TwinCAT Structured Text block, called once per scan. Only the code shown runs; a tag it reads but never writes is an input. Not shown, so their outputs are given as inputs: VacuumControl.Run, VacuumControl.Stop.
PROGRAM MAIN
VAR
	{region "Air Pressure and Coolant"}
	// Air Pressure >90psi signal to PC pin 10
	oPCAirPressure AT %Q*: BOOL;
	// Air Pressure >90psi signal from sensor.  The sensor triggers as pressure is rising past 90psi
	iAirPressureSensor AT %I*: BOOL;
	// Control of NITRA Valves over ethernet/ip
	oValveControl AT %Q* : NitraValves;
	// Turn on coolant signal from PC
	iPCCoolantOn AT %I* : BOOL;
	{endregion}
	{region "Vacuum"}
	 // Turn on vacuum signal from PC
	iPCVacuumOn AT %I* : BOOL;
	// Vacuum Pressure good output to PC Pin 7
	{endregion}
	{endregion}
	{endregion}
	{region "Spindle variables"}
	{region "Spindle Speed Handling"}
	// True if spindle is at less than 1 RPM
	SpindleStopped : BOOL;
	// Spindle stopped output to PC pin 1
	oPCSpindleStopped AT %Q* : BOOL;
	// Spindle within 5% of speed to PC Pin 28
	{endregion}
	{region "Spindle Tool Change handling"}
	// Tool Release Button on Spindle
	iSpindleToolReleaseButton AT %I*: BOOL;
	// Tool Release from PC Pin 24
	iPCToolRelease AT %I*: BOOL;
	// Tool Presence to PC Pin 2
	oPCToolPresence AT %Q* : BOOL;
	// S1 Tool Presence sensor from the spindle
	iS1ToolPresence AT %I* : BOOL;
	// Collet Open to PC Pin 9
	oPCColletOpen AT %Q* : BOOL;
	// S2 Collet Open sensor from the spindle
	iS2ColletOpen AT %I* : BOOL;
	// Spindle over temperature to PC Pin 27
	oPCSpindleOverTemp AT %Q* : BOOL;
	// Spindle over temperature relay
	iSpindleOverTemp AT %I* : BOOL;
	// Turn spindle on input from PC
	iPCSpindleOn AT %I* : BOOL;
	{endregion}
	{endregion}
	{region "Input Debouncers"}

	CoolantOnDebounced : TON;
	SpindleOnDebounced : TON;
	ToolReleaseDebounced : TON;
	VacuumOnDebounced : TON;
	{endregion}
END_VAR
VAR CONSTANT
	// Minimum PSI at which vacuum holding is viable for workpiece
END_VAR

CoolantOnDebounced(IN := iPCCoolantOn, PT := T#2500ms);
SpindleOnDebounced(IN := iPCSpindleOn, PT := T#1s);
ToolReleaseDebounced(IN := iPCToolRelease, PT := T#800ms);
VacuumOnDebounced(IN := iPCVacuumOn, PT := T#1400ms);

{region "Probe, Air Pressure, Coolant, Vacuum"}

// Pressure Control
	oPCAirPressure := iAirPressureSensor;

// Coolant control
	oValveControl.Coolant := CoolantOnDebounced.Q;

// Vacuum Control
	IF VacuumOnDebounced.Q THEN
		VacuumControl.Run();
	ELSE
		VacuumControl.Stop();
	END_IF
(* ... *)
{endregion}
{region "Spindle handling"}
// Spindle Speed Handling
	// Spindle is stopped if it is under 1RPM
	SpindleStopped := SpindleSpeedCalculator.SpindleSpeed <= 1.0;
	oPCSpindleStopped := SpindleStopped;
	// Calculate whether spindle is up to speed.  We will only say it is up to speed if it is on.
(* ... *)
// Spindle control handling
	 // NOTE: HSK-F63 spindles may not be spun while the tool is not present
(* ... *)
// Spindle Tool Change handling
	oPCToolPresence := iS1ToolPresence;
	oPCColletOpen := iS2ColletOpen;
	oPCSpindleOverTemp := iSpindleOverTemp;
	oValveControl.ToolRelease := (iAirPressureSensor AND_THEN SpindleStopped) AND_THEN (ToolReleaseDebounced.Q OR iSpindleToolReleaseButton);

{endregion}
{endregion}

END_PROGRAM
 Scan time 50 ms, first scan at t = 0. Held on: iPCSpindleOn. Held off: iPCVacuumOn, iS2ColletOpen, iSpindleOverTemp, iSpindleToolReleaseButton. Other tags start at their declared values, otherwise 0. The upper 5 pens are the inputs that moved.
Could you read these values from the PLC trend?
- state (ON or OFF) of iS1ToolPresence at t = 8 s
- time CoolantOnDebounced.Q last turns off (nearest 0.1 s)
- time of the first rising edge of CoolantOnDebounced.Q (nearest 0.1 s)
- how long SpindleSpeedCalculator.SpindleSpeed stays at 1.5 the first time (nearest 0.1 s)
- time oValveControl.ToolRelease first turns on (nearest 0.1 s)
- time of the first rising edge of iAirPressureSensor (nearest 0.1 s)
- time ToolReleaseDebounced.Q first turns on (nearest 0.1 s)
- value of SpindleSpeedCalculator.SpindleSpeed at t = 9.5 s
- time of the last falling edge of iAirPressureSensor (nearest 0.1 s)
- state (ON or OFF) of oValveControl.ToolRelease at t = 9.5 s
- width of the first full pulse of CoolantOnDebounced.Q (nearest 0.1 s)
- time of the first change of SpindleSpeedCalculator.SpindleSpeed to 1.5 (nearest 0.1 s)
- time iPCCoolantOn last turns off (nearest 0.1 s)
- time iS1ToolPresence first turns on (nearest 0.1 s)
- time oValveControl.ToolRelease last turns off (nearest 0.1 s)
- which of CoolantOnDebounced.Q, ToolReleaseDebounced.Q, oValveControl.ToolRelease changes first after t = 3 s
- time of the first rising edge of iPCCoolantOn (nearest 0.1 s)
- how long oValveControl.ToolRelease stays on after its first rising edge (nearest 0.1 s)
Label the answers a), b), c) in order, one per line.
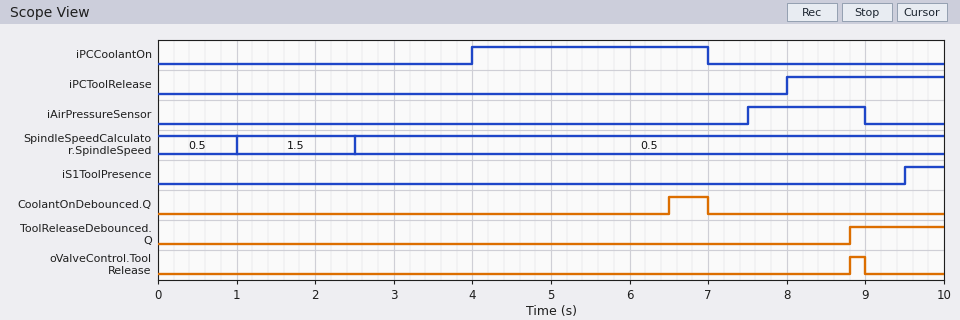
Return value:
a) OFF
b) 7.0 s
c) 6.5 s
d) 1.5 s
e) 8.8 s
f) 7.5 s
g) 8.8 s
h) 0.5
i) 9.0 s
j) OFF
k) 0.5 s
l) 1.0 s
m) 7.0 s
n) 9.5 s
o) 9.0 s
p) CoolantOnDebounced.Q
q) 4.0 s
r) 0.2 s
